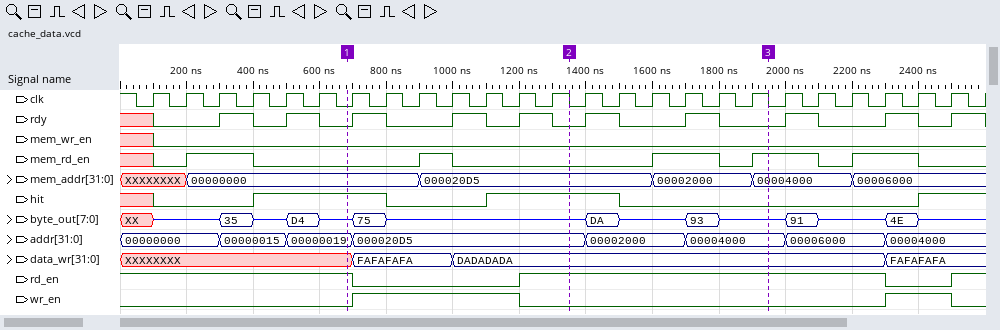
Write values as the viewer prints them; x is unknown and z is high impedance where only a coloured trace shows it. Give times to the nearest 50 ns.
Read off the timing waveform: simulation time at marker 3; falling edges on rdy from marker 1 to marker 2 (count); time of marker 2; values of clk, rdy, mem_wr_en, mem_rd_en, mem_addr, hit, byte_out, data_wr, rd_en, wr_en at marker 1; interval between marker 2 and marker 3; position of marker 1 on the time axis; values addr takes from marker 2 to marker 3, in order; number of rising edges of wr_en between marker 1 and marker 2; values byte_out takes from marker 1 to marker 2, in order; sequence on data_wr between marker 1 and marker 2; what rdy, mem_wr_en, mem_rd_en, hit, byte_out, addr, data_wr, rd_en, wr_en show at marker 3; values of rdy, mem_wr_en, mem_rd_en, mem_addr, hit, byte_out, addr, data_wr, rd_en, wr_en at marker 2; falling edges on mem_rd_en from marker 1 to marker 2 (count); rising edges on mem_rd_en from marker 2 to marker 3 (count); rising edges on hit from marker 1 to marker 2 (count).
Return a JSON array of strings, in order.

["1950 ns", "3", "1350 ns", "clk=0, rdy=0, mem_wr_en=0, mem_rd_en=0, mem_addr=00000000, hit=1, byte_out=z, data_wr=XXXXXXXX, rd_en=1, wr_en=0", "600 ns", "700 ns", "000020D5, 00002000, 00004000", "1", "z, 75, z", "XXXXXXXX, FAFAFAFA, DADADADA", "rdy=0, mem_wr_en=0, mem_rd_en=1, hit=0, byte_out=z, addr=00004000, data_wr=DADADADA, rd_en=1, wr_en=0", "rdy=0, mem_wr_en=0, mem_rd_en=0, mem_addr=000020D5, hit=1, byte_out=z, addr=000020D5, data_wr=DADADADA, rd_en=1, wr_en=0", "1", "2", "1"]
